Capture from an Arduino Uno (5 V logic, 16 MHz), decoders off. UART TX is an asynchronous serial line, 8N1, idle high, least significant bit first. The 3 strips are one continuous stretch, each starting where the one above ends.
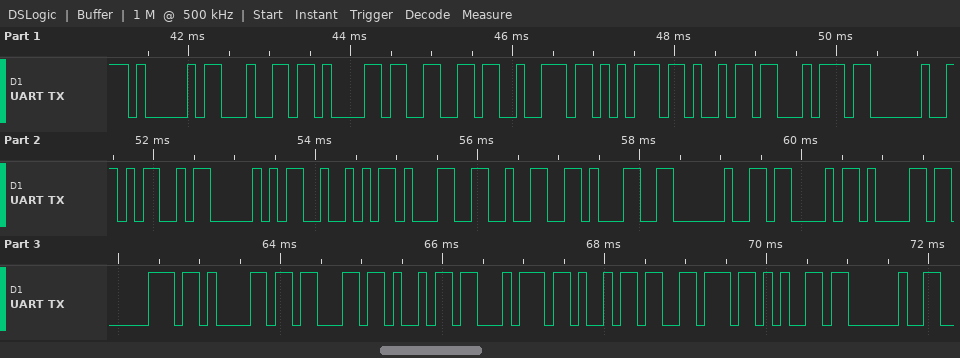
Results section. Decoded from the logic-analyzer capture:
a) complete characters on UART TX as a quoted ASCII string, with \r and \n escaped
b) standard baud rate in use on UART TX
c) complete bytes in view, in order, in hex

"Adafruit MPR121 Capacitive "
9600 baud
41 64 61 66 72 75 69 74 20 4D 50 52 31 32 31 20 43 61 70 61 63 69 74 69 76 65 20
